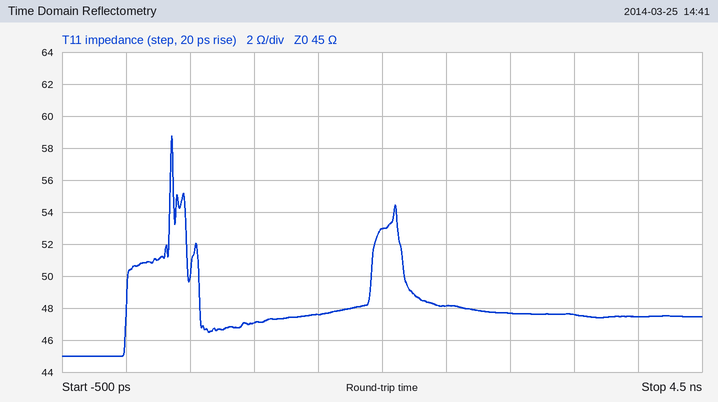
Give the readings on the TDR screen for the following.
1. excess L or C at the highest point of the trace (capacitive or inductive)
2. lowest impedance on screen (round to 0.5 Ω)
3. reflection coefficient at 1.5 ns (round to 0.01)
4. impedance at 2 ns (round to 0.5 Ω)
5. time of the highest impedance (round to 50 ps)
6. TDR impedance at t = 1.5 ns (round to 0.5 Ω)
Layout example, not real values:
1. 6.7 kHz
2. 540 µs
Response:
1. inductive
2. 45.0 Ω
3. +0.03
4. 53.0 Ω
5. 350 ps
6. 47.5 Ω
